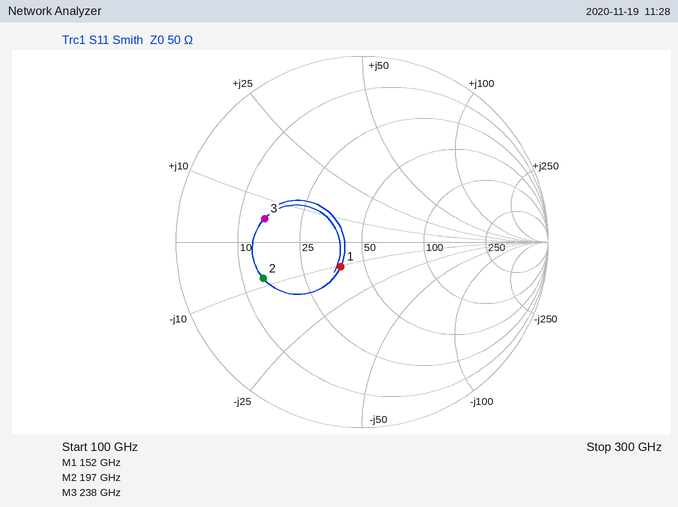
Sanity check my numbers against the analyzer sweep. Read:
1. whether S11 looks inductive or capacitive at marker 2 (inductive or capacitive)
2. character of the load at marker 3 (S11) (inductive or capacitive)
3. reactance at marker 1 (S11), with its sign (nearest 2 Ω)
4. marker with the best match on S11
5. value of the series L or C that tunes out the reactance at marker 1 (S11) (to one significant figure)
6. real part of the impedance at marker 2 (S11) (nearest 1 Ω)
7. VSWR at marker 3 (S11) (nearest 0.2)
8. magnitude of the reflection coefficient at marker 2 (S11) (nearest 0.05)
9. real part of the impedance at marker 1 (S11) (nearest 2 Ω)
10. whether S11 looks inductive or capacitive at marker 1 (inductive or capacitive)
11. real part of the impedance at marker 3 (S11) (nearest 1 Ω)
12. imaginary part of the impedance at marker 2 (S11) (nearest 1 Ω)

capacitive
inductive
-10 Ω
marker 1
10 pH
14 Ω
3.4
0.55
38 Ω
capacitive
15 Ω
-8 Ω
